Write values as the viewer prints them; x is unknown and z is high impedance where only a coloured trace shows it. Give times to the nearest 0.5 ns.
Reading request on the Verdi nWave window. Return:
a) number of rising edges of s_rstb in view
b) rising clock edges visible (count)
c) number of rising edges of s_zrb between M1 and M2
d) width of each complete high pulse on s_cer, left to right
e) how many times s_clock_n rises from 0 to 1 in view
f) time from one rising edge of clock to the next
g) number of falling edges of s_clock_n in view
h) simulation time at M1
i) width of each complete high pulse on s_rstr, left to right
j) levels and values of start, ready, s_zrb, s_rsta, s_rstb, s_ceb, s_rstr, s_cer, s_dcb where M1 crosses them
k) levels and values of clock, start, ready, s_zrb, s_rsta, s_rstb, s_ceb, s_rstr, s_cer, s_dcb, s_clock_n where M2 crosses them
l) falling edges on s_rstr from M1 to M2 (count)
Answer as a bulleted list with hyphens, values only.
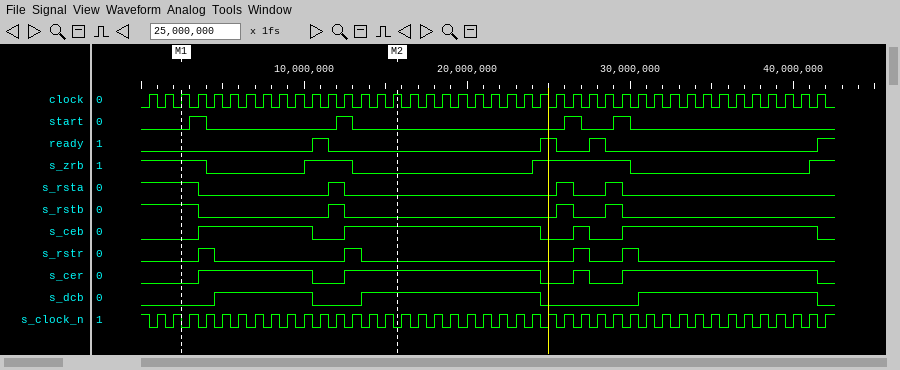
- 3
- 42
- 1
- 7 ns, 12 ns, 1 ns, 12 ns
- 42
- 1 ns
- 42
- 2.5 ns
- 1 ns, 1 ns, 1 ns, 1 ns
- start=0, ready=0, s_zrb=1, s_rsta=1, s_rstb=1, s_ceb=0, s_rstr=0, s_cer=0, s_dcb=0
- clock=1, start=0, ready=0, s_zrb=0, s_rsta=0, s_rstb=0, s_ceb=1, s_rstr=0, s_cer=1, s_dcb=1, s_clock_n=0
- 2
